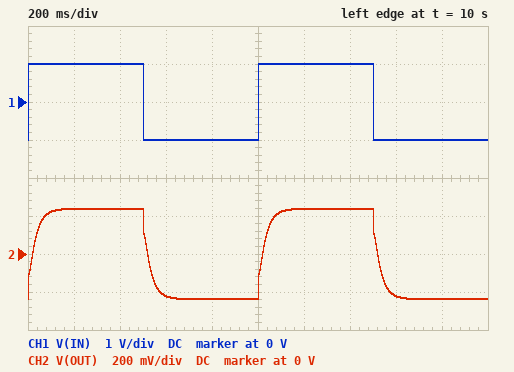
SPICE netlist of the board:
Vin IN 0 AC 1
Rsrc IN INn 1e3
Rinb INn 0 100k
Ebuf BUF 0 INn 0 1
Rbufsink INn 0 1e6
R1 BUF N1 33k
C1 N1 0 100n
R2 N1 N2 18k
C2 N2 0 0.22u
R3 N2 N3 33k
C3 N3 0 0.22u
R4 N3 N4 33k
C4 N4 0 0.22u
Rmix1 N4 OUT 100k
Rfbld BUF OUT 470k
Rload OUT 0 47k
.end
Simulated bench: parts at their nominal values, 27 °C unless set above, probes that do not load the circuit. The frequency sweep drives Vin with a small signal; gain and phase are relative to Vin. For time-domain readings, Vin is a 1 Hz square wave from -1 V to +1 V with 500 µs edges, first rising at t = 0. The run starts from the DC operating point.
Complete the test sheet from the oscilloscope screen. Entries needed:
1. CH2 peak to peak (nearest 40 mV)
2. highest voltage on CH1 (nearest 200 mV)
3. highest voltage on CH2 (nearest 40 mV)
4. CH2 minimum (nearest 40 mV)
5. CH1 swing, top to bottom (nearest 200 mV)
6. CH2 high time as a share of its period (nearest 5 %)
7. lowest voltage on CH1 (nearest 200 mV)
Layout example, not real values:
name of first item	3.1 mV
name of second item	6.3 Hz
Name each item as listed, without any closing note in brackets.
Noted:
CH2 peak to peak	480 mV
highest voltage on CH1	1.0 V
highest voltage on CH2	240 mV
CH2 minimum	-240 mV
CH1 swing, top to bottom	2.0 V
CH2 high time as a share of its period	50 %
lowest voltage on CH1	-1.0 V
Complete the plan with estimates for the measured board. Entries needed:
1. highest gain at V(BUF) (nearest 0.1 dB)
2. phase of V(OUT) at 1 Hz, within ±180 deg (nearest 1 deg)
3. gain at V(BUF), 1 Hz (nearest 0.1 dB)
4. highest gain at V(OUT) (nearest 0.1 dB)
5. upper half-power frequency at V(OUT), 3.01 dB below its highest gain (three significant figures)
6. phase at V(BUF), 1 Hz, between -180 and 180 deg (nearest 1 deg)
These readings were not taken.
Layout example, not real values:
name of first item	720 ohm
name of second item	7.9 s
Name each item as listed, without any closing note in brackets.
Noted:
highest gain at V(BUF)	-0.1 dB
phase of V(OUT) at 1 Hz, within ±180 deg	-10 deg
gain at V(BUF), 1 Hz	-0.1 dB
highest gain at V(OUT)	-12.5 dB
upper half-power frequency at V(OUT), 3.01 dB below its highest gain	5.00 Hz
phase at V(BUF), 1 Hz, between -180 and 180 deg	0 deg
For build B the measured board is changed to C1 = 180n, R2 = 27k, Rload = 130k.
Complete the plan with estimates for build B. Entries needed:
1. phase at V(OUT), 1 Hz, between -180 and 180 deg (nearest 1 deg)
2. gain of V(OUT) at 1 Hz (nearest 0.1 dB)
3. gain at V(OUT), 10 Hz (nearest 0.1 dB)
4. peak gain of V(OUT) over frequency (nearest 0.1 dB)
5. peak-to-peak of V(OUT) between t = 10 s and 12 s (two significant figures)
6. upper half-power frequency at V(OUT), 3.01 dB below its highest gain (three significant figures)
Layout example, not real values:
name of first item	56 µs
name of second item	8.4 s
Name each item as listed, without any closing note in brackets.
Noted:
phase at V(OUT), 1 Hz, between -180 and 180 deg	-12 deg
gain of V(OUT) at 1 Hz	-7.1 dB
gain at V(OUT), 10 Hz	-16.4 dB
peak gain of V(OUT) over frequency	-6.8 dB
peak-to-peak of V(OUT) between t = 10 s and 12 s	910 mV
upper half-power frequency at V(OUT), 3.01 dB below its highest gain	4.02 Hz
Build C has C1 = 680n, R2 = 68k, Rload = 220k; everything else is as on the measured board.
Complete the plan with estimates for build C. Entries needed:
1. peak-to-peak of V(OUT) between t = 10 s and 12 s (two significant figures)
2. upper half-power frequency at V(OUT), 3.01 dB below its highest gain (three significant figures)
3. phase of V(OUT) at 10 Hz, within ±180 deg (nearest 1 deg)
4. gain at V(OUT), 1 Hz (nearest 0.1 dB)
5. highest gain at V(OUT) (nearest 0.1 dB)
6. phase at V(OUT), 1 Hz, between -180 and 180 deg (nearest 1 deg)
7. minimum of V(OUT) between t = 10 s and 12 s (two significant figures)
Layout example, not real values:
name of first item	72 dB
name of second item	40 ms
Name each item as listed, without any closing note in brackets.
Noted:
peak-to-peak of V(OUT) between t = 10 s and 12 s	1.1 V
upper half-power frequency at V(OUT), 3.01 dB below its highest gain	2.49 Hz
phase of V(OUT) at 10 Hz, within ±180 deg	-34 deg
gain at V(OUT), 1 Hz	-5.7 dB
highest gain at V(OUT)	-5.1 dB
phase at V(OUT), 1 Hz, between -180 and 180 deg	-20 deg
minimum of V(OUT) between t = 10 s and 12 s	-560 mV
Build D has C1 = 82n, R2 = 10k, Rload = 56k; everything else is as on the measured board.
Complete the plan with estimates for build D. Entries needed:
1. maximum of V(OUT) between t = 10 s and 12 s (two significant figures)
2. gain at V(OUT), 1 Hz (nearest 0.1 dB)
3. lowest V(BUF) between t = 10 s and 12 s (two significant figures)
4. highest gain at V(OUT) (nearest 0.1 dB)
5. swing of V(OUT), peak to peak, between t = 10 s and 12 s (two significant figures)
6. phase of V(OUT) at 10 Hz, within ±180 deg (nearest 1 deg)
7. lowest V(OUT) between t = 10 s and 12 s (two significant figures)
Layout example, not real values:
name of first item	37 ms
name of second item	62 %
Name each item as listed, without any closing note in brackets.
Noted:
maximum of V(OUT) between t = 10 s and 12 s	280 mV
gain at V(OUT), 1 Hz	-11.3 dB
lowest V(BUF) between t = 10 s and 12 s	-990 mV
highest gain at V(OUT)	-11.2 dB
swing of V(OUT), peak to peak, between t = 10 s and 12 s	550 mV
phase of V(OUT) at 10 Hz, within ±180 deg	-51 deg
lowest V(OUT) between t = 10 s and 12 s	-280 mV
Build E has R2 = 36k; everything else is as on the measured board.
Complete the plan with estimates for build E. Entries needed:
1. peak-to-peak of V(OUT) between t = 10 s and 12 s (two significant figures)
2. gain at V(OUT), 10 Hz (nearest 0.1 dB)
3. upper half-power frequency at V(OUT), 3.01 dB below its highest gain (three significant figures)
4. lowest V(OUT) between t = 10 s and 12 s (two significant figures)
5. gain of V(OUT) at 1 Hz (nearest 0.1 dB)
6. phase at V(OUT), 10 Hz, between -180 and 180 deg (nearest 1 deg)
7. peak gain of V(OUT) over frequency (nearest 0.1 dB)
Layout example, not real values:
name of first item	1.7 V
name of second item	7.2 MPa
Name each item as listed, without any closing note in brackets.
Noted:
peak-to-peak of V(OUT) between t = 10 s and 12 s	460 mV
gain at V(OUT), 10 Hz	-21.3 dB
upper half-power frequency at V(OUT), 3.01 dB below its highest gain	4.41 Hz
lowest V(OUT) between t = 10 s and 12 s	-230 mV
gain of V(OUT) at 1 Hz	-13.0 dB
phase at V(OUT), 10 Hz, between -180 and 180 deg	-48 deg
peak gain of V(OUT) over frequency	-12.8 dB
